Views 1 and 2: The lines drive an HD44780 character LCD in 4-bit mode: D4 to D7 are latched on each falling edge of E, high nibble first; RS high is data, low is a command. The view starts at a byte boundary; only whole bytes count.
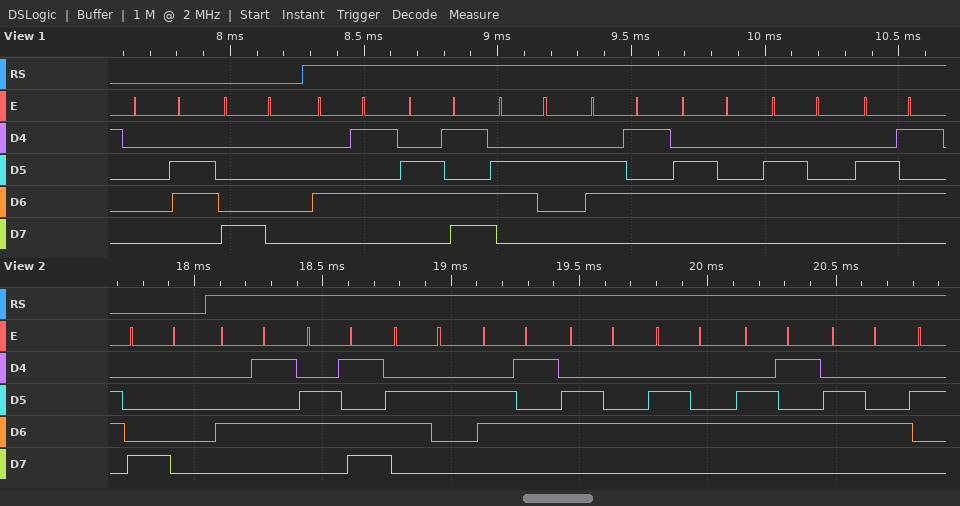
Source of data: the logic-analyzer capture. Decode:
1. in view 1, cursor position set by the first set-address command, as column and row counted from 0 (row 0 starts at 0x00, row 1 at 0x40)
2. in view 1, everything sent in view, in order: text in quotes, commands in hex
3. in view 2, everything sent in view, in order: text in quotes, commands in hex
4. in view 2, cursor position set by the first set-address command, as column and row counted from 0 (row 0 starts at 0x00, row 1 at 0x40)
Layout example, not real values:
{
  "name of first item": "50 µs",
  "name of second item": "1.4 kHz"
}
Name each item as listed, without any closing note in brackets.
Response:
{
  "in view 1, cursor position set by the first set-address command, as column and row counted from 0": "column 0, row 0",
  "in view 1, everything sent in view, in order: text in quotes, commands in hex": "0x06 0x80 \"Embedde\"",
  "in view 2, everything sent in view, in order: text in quotes, commands in hex": "0x80 \"Embedded\"",
  "in view 2, cursor position set by the first set-address command, as column and row counted from 0": "column 0, row 0"
}
